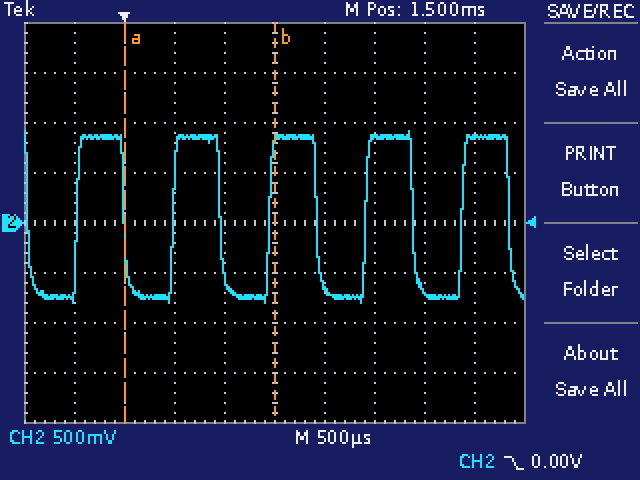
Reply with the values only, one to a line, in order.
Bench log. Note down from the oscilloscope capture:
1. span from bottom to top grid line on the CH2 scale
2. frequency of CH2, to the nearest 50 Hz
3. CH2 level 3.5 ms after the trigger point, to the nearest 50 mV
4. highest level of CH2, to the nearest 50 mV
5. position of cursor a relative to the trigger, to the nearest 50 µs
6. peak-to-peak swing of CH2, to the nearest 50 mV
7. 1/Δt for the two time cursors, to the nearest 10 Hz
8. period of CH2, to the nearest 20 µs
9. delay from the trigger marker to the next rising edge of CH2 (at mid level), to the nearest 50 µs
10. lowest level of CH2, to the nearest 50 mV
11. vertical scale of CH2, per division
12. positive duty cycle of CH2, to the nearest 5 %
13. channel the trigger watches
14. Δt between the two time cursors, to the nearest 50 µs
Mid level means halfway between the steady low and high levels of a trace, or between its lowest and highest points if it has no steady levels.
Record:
4 V
1.05 kHz
850 mV
900 mV
0 µs
1.70 V
670 Hz
960 µs
500 µs
-800 mV
500 mV
50 %
CH2
1.50 ms
